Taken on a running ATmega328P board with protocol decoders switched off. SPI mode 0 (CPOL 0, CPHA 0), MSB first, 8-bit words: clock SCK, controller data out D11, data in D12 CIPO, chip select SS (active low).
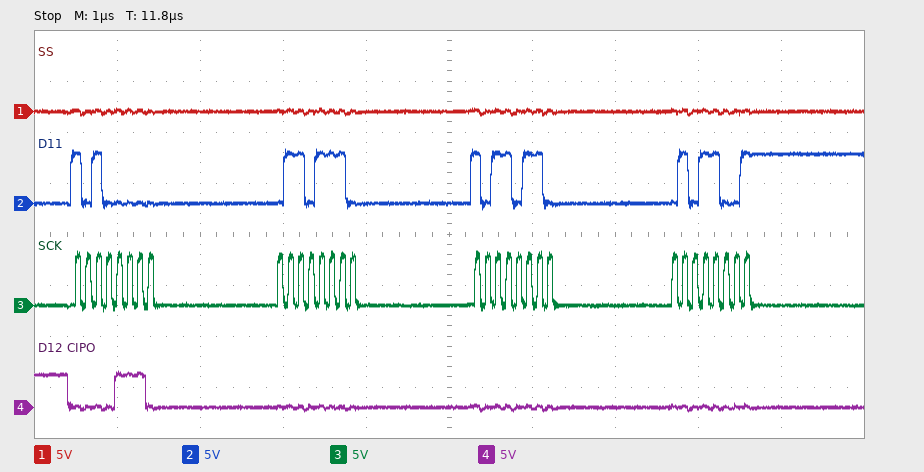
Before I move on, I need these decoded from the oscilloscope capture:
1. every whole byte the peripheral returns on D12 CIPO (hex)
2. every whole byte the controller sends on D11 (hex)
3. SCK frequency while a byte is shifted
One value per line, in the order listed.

0E 00 00 00
A0 6E B6 59
8 MHz
